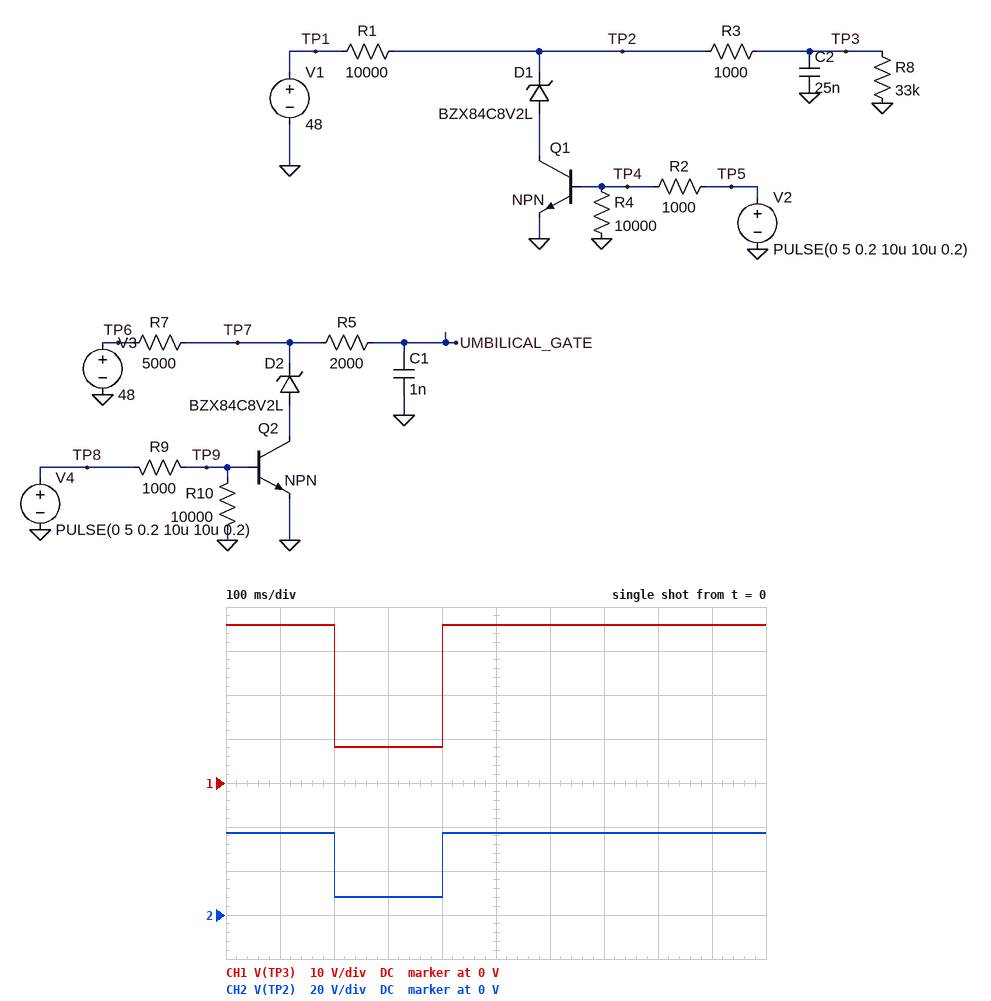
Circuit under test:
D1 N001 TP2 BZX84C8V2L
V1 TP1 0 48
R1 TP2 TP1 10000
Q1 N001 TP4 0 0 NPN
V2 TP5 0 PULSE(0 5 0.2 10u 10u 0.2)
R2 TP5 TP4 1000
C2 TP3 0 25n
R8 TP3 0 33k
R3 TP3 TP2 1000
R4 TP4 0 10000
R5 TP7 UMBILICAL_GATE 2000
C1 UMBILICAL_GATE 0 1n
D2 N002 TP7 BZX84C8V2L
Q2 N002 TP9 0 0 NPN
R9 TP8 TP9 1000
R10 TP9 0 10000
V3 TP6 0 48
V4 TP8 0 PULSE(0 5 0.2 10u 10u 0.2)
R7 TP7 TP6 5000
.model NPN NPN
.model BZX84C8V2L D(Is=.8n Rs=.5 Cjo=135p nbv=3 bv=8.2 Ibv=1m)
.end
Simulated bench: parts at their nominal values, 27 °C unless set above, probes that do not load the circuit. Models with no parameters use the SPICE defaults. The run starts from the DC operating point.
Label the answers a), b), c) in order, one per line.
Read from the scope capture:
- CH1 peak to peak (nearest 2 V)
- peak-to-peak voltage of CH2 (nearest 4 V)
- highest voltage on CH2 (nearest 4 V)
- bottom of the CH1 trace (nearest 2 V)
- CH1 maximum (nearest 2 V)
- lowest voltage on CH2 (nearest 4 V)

a) 28 V
b) 28 V
c) 36 V
d) 8 V
e) 36 V
f) 8 V
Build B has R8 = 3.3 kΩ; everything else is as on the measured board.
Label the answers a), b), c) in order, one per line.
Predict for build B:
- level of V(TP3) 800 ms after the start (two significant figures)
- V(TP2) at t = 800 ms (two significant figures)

a) 11 V
b) 14 V
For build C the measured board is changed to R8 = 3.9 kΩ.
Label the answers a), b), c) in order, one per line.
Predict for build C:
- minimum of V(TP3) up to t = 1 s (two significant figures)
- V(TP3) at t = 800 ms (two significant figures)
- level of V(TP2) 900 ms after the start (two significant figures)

a) 6.6 V
b) 13 V
c) 16 V
